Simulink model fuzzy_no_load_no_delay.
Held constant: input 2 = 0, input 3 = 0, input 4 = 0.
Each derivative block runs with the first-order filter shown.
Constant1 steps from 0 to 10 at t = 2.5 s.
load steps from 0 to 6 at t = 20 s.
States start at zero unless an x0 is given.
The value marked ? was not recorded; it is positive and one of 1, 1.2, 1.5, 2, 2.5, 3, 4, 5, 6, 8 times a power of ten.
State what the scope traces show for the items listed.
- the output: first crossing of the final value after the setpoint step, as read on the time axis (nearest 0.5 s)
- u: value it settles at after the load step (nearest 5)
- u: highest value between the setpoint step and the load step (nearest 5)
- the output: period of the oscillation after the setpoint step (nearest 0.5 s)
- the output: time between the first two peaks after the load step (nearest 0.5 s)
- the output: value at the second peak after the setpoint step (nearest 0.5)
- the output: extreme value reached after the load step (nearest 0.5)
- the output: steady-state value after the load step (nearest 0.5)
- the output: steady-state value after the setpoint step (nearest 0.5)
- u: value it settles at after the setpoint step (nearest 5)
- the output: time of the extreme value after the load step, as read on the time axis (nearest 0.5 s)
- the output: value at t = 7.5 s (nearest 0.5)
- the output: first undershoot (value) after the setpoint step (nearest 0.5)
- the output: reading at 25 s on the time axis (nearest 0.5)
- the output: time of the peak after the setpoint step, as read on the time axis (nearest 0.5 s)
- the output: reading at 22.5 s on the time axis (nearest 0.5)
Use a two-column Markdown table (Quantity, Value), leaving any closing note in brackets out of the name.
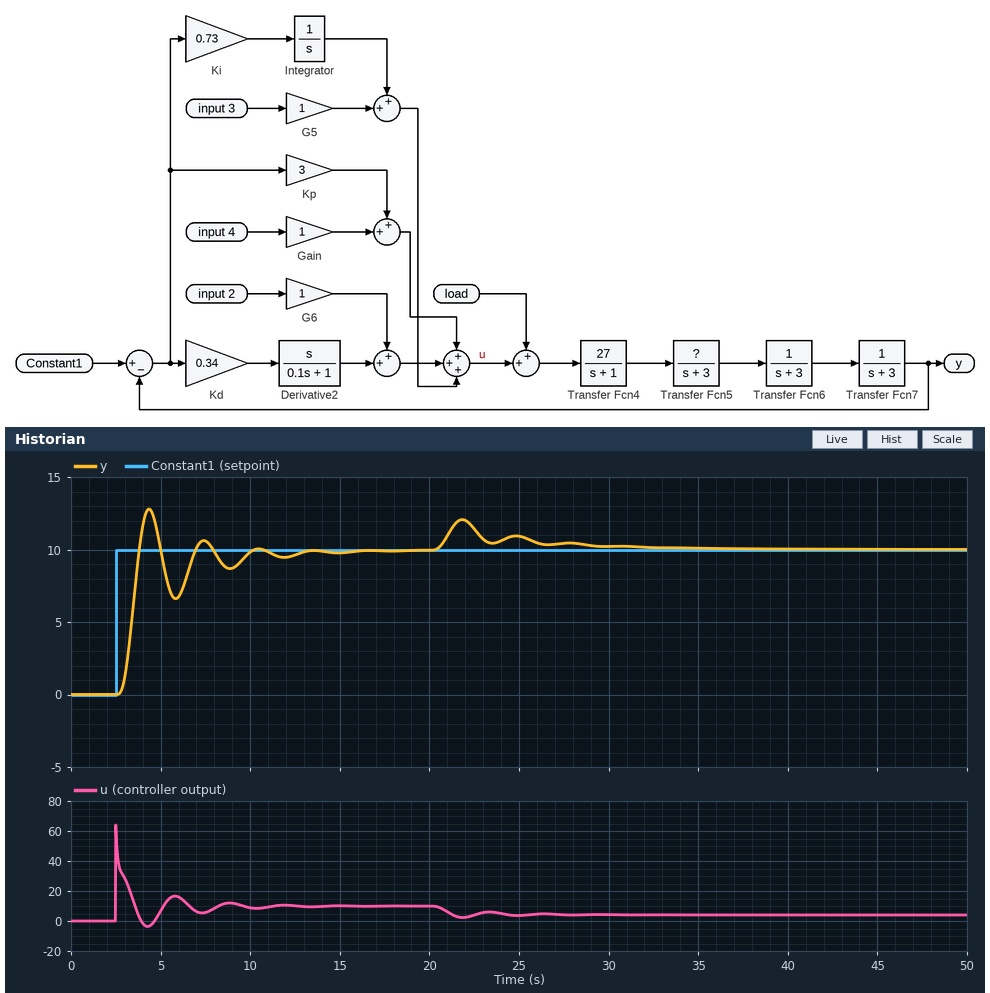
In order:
| Quantity | Value |
|---|---|
| the output: first crossing of the final value after the setpoint step, as read on the time axis | 4.0 s |
| u: value it settles at after the load step | 5 |
| u: highest value between the setpoint step and the load step | 65 |
| the output: period of the oscillation after the setpoint step | 3.0 s |
| the output: time between the first two peaks after the load step | 3.0 s |
| the output: value at the second peak after the setpoint step | 10.5 |
| the output: extreme value reached after the load step | 12.0 |
| the output: steady-state value after the load step | 10.0 |
| the output: steady-state value after the setpoint step | 10.0 |
| u: value it settles at after the setpoint step | 10 |
| the output: time of the extreme value after the load step, as read on the time axis | 22.0 s |
| the output: value at t = 7.5 s | 10.5 |
| the output: first undershoot (value) after the setpoint step | 6.5 |
| the output: reading at 25 s on the time axis | 11.0 |
| the output: time of the peak after the setpoint step, as read on the time axis | 4.5 s |
| the output: reading at 22.5 s on the time axis | 11.5 |
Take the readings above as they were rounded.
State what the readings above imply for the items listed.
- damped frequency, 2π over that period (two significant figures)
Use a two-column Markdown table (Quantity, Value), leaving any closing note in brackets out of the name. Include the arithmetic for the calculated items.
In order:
| Quantity | Value |
|---|---|
| damped frequency, 2π over that period | 2π / 3 = 2.1 rad/s |
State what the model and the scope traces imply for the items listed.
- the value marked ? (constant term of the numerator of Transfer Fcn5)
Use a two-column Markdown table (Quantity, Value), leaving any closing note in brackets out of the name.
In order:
| Quantity | Value |
|---|---|
| the value marked ? | 1 |
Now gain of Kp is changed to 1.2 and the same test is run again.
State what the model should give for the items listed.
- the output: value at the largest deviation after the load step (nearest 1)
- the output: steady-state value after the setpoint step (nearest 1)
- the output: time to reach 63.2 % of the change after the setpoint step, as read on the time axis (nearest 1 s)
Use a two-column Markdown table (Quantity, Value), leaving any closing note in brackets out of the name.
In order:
| Quantity | Value |
|---|---|
| the output: value at the largest deviation after the load step | 13 |
| the output: steady-state value after the setpoint step | 10 |
| the output: time to reach 63.2 % of the change after the setpoint step, as read on the time axis | 4 s |
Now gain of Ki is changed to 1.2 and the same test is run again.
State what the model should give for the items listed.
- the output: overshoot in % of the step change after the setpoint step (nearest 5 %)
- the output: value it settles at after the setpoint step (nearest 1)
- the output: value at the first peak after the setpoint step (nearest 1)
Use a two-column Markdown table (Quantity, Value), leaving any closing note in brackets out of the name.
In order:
| Quantity | Value |
|---|---|
| the output: overshoot in % of the step change after the setpoint step | 40 % |
| the output: value it settles at after the setpoint step | 10 |
| the output: value at the first peak after the setpoint step | 14 |
